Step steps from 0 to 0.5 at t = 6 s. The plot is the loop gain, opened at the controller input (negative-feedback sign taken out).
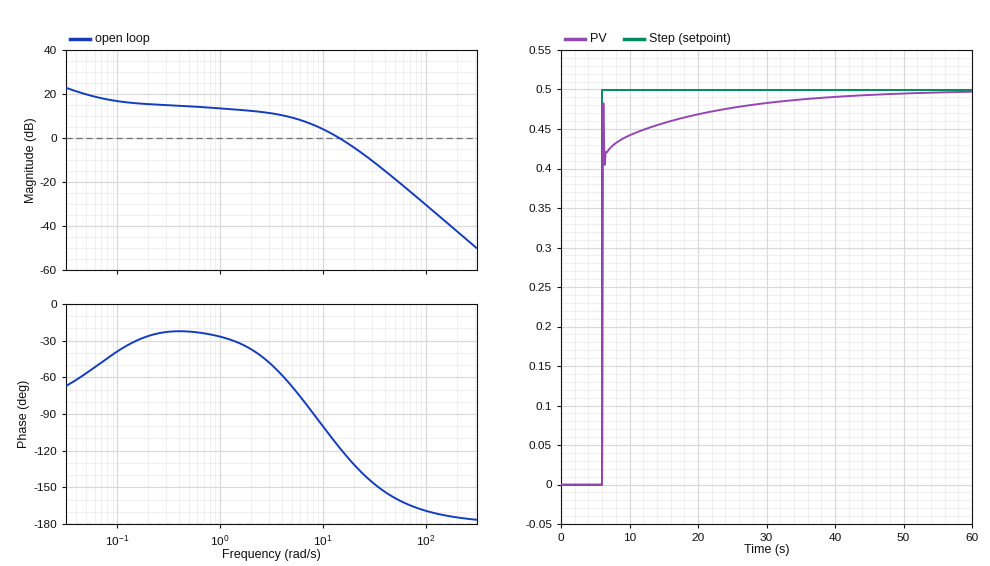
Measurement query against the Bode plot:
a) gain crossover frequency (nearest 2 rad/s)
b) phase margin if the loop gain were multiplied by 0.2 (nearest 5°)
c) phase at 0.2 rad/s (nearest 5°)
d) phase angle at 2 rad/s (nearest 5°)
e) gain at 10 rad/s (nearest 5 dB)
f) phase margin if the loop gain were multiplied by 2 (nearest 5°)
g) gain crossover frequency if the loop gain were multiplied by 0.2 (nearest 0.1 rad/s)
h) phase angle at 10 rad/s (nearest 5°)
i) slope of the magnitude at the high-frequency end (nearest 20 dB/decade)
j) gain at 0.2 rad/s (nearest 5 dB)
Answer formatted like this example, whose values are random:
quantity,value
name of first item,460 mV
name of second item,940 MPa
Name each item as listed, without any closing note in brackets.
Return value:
quantity,value
gain crossover frequency,14 rad/s
phase margin if the loop gain were multiplied by 0.2,155°
phase at 0.2 rad/s,-25°
phase angle at 2 rad/s,-35°
gain at 10 rad/s,5 dB
phase margin if the loop gain were multiplied by 2,45°
gain crossover frequency if the loop gain were multiplied by 0.2,0.7 rad/s
phase angle at 10 rad/s,-100°
slope of the magnitude at the high-frequency end,-40 dB/decade
gain at 0.2 rad/s,15 dB
